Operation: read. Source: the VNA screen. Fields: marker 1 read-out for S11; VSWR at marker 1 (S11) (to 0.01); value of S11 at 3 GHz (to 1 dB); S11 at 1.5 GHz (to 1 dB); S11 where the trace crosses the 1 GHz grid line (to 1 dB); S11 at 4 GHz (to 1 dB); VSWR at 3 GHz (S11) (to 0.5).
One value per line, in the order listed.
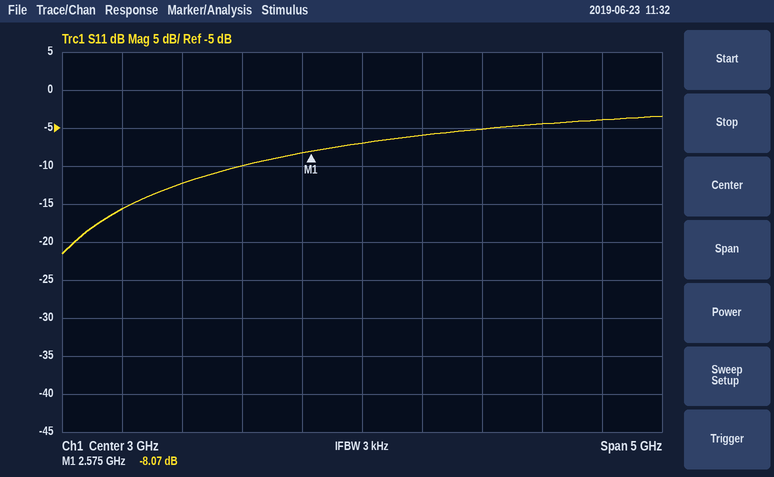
-8.07 dB
2.31
-7 dB
-12 dB
-16 dB
-5 dB
2.5
